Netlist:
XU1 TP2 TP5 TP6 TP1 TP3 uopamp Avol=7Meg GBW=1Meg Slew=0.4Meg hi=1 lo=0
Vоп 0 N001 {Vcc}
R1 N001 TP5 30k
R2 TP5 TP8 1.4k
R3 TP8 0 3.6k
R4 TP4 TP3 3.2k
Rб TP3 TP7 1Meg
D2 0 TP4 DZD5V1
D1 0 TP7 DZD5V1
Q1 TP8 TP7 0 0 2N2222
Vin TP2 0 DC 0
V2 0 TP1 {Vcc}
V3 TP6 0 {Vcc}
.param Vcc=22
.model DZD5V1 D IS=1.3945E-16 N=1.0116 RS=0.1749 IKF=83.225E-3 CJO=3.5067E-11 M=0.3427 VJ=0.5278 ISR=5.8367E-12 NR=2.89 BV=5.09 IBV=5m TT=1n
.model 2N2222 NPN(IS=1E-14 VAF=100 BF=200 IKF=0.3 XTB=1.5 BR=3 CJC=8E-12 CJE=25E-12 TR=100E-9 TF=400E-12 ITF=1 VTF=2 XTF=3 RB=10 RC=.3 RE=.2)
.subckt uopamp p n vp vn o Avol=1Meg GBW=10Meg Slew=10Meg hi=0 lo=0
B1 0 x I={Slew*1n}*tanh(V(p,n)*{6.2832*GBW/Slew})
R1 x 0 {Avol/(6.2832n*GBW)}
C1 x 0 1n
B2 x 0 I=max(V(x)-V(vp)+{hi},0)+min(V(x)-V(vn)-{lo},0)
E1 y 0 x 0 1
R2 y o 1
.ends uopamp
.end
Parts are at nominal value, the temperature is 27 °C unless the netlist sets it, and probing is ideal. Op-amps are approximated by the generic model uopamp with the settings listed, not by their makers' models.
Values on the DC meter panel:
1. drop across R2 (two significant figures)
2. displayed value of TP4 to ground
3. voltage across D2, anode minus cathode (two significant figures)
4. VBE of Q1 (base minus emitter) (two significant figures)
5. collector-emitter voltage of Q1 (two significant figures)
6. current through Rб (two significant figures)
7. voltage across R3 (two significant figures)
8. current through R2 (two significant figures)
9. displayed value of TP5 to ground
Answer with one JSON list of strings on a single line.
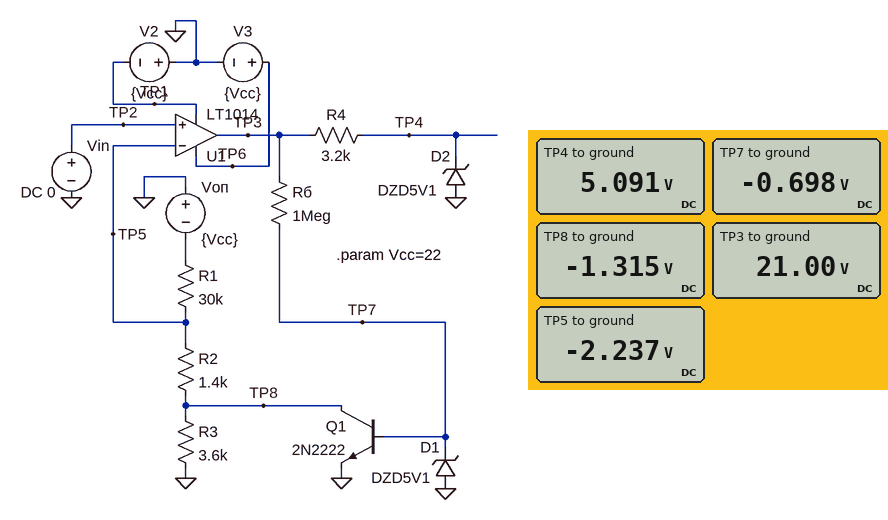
["920 mV", "5.091 V", "-5.1 V", "-700 mV", "-1.3 V", "22 µA", "1.3 V", "660 µA", "-2.237 V"]
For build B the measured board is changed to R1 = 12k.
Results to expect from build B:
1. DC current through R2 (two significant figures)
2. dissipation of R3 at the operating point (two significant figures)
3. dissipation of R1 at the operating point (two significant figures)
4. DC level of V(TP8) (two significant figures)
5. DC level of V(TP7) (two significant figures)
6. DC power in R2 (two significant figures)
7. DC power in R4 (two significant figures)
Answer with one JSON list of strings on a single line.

["1.5 mA", "540 µW", "28 mW", "-1.4 V", "-740 mV", "3.3 mW", "79 mW"]
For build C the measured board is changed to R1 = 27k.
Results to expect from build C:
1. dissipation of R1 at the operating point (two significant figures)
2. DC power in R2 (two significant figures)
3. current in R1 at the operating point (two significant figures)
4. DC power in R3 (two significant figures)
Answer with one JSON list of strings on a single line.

["14 mW", "740 µW", "730 µA", "490 µW"]
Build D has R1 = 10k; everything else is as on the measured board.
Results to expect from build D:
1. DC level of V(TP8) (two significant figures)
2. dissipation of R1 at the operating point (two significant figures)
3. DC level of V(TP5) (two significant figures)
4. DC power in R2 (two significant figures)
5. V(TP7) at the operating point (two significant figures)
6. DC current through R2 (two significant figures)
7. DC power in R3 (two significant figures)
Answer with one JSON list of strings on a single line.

["-1.4 V", "33 mW", "-3.9 V", "4.6 mW", "-750 mV", "1.8 mA", "550 µW"]
